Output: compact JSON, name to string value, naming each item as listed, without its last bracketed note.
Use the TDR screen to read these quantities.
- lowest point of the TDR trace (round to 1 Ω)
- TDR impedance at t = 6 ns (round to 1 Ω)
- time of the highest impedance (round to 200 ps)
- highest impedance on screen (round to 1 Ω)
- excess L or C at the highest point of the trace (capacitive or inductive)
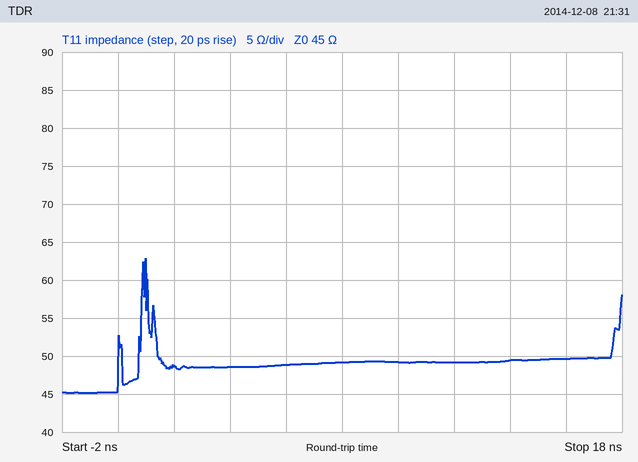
{"lowest point of the TDR trace": "45 Ω", "TDR impedance at t = 6 ns": "49 Ω", "time of the highest impedance": "1.0 ns", "highest impedance on screen": "63 Ω", "excess L or C at the highest point of the trace": "inductive"}
